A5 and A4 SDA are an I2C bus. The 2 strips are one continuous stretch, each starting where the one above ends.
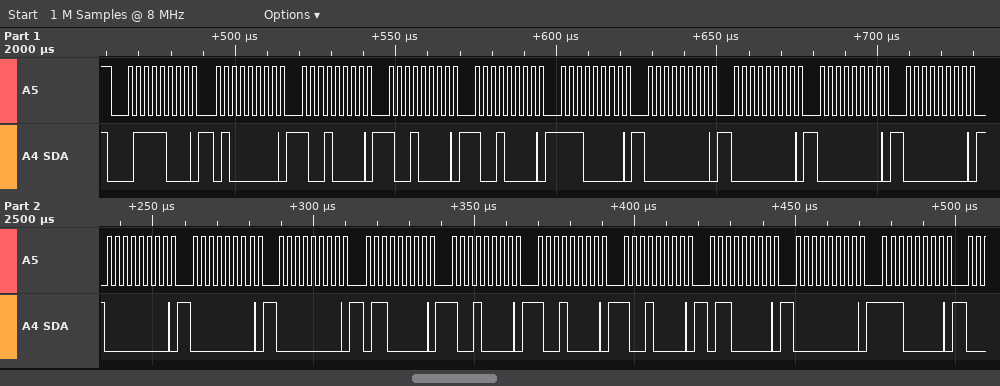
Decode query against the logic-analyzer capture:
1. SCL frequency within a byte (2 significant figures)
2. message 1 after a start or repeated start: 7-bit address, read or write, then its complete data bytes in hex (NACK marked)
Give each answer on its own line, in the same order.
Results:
400 kHz
0x3C write: 40 90 90 90 E0 00 00 00 00 00 00 00 60 90 90 90 60 00 E0
